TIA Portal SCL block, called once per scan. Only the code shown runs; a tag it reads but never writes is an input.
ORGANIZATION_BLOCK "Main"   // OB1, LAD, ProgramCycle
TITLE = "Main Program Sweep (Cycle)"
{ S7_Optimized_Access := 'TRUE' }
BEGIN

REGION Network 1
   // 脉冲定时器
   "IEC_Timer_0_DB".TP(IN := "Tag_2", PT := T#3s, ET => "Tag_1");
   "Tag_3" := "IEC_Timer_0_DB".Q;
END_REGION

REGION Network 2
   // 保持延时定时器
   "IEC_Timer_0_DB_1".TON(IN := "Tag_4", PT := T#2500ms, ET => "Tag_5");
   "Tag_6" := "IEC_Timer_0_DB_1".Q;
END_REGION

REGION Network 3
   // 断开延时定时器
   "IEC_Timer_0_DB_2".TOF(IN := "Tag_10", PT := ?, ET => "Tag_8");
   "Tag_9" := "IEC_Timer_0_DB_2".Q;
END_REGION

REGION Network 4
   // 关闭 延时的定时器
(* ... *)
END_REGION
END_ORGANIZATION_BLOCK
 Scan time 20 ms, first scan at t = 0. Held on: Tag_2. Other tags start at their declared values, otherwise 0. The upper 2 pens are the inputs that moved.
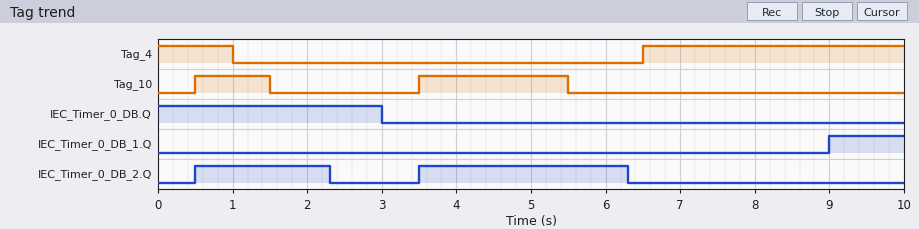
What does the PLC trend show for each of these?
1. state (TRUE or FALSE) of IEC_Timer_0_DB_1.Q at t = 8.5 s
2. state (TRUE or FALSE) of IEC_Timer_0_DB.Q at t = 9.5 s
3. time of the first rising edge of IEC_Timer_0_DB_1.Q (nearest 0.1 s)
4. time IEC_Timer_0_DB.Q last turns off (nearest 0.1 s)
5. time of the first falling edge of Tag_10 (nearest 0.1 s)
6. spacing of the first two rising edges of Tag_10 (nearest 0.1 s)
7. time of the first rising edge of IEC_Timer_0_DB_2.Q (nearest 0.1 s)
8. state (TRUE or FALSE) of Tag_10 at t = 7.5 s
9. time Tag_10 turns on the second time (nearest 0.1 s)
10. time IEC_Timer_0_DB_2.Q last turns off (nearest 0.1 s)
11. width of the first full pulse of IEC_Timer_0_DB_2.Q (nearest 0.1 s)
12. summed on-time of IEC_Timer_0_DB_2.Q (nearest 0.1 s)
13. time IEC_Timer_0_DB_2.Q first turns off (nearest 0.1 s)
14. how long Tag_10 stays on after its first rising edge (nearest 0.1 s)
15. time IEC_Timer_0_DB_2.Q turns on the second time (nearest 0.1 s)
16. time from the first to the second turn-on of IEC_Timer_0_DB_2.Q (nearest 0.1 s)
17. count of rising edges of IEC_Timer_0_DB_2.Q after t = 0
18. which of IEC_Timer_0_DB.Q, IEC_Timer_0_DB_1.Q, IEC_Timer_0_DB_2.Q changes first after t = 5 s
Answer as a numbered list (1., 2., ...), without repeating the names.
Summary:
1. FALSE
2. FALSE
3. 9.0 s
4. 3.0 s
5. 1.5 s
6. 3.0 s
7. 0.5 s
8. FALSE
9. 3.5 s
10. 6.3 s
11. 1.8 s
12. 4.6 s
13. 2.3 s
14. 1.0 s
15. 3.5 s
16. 3.0 s
17. 2
18. IEC_Timer_0_DB_2.Q
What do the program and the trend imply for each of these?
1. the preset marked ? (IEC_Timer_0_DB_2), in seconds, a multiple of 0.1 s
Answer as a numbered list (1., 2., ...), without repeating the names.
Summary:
1. 0.8 s
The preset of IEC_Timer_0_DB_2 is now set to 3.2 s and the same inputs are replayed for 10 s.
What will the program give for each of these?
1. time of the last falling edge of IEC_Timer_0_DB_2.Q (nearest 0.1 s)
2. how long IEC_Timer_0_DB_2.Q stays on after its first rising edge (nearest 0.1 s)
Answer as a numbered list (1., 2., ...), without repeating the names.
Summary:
1. 8.7 s
2. 8.2 s
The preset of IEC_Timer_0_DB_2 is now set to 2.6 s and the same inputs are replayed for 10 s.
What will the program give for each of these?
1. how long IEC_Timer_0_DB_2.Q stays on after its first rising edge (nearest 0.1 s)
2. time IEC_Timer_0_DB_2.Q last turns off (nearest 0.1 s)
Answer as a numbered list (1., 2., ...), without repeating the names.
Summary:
1. 7.6 s
2. 8.1 s
